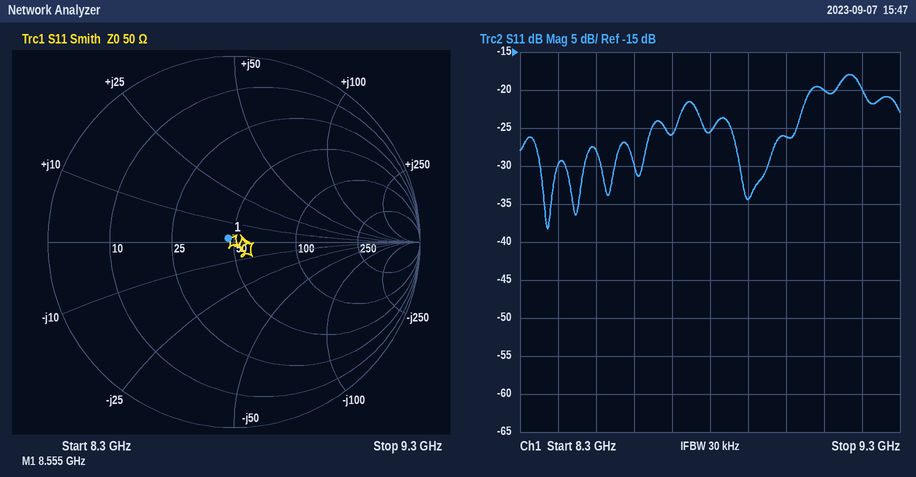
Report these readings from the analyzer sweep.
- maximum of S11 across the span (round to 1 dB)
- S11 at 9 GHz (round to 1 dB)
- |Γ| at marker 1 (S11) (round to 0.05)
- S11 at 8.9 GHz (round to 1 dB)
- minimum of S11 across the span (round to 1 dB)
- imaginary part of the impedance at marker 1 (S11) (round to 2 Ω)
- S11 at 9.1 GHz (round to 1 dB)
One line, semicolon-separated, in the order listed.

-18 dB; -26 dB; 0.05; -34 dB; -38 dB; +2 Ω; -20 dB
